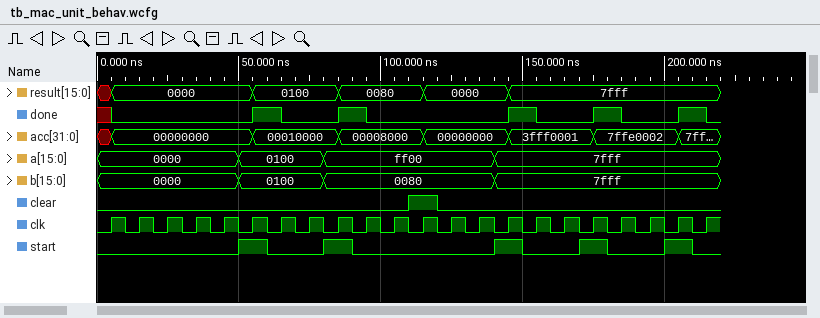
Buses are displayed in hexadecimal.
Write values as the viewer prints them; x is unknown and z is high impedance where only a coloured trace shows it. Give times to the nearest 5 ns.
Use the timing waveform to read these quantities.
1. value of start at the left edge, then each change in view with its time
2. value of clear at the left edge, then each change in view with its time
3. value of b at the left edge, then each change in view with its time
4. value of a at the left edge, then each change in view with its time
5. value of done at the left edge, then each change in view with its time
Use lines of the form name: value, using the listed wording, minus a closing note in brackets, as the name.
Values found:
value of start at the left edge, then each change in view with its time: 0, 1 at 50 ns, 0 at 60 ns, 1 at 80 ns, 0 at 90 ns, 1 at 140 ns, 0 at 150 ns, 1 at 170 ns, 0 at 180 ns, 1 at 200 ns, 0 at 210 ns
value of clear at the left edge, then each change in view with its time: 0, 1 at 110 ns, 0 at 120 ns
value of b at the left edge, then each change in view with its time: 0000, 0100 at 50 ns, 0080 at 80 ns, 7fff at 140 ns
value of a at the left edge, then each change in view with its time: 0000, 0100 at 50 ns, ff00 at 80 ns, 7fff at 140 ns
value of done at the left edge, then each change in view with its time: x, 0 at 5 ns, 1 at 55 ns, 0 at 65 ns, 1 at 85 ns, 0 at 95 ns, 1 at 145 ns, 0 at 155 ns, 1 at 175 ns, 0 at 185 ns, 1 at 205 ns, 0 at 215 ns
